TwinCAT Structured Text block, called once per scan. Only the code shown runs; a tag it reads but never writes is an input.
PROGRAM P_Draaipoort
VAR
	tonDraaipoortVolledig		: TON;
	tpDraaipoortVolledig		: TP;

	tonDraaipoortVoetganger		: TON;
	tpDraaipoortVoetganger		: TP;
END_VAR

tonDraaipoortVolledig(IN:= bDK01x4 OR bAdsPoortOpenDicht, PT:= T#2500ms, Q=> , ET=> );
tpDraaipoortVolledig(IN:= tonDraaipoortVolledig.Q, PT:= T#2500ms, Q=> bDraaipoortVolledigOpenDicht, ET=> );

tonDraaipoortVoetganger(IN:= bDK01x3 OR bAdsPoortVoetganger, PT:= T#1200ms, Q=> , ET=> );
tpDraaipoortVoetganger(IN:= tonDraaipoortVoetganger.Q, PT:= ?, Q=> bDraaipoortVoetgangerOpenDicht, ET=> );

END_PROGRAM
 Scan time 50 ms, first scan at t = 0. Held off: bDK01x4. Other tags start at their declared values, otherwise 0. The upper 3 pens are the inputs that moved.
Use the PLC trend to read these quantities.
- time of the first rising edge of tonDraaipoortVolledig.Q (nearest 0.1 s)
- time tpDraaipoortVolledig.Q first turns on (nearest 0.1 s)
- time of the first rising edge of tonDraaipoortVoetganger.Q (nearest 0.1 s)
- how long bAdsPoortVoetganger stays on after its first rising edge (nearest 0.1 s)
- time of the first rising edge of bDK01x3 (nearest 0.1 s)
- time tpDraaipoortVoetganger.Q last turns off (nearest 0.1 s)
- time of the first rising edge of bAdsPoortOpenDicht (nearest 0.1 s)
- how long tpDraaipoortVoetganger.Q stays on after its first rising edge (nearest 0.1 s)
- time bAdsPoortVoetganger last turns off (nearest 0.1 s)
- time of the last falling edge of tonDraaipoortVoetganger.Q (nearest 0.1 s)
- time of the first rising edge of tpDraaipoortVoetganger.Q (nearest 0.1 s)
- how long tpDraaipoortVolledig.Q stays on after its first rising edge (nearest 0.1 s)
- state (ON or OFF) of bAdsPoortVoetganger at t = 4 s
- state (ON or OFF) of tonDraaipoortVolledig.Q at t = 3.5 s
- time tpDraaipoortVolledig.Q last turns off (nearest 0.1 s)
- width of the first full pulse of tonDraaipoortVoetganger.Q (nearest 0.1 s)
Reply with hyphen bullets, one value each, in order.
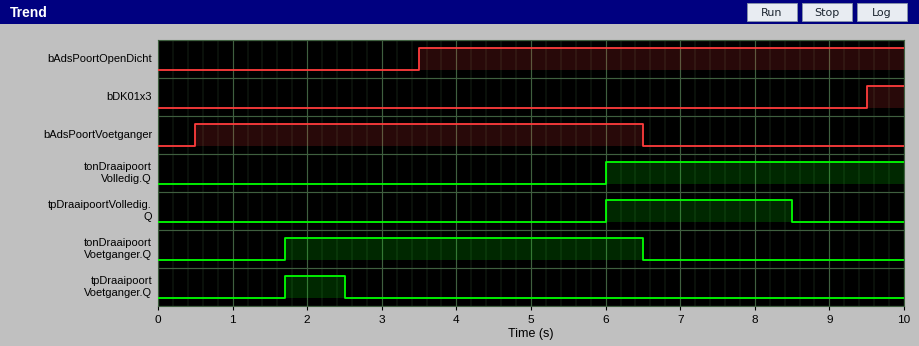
- 6.0 s
- 6.0 s
- 1.7 s
- 6.0 s
- 9.5 s
- 2.5 s
- 3.5 s
- 0.8 s
- 6.5 s
- 6.5 s
- 1.7 s
- 2.5 s
- ON
- OFF
- 8.5 s
- 4.8 s
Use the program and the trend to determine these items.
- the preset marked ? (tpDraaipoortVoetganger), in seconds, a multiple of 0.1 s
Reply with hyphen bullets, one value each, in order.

- 0.8 s
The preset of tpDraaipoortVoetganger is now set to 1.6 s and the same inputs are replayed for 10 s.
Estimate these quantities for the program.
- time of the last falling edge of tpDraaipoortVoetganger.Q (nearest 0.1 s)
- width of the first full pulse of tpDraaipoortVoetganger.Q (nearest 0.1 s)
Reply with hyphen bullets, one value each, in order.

- 3.3 s
- 1.6 s
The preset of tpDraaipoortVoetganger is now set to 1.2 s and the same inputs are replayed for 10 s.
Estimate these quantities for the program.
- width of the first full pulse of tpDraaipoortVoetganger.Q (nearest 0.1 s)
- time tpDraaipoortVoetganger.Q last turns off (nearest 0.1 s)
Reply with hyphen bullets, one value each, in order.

- 1.2 s
- 2.9 s
